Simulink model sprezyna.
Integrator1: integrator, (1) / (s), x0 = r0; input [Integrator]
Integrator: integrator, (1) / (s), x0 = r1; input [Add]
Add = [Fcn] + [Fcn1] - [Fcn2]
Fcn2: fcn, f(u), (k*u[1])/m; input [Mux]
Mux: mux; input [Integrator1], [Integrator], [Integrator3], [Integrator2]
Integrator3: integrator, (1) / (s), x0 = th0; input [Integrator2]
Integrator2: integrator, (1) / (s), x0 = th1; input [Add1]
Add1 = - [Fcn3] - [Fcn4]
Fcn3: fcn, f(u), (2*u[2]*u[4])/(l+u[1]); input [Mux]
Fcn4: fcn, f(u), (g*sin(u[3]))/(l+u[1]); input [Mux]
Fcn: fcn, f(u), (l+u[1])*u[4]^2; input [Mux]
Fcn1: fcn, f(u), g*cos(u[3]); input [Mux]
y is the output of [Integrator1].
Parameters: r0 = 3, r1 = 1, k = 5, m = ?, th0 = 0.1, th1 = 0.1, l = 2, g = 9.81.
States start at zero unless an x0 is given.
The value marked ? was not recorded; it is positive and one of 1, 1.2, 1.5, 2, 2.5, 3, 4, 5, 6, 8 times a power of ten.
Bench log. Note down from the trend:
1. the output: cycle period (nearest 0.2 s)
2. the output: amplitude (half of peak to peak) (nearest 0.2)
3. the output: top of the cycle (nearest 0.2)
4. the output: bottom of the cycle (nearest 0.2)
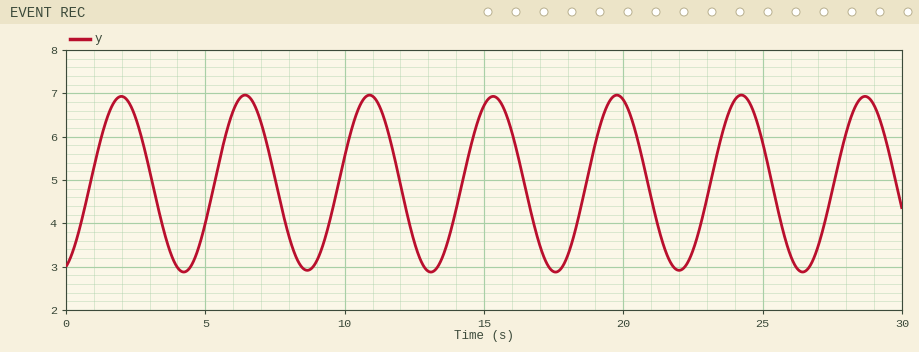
4.4 s
2.0
7.0
2.8
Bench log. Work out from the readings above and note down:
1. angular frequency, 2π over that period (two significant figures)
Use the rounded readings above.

1.4 rad/s
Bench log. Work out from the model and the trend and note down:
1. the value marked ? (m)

2.5
